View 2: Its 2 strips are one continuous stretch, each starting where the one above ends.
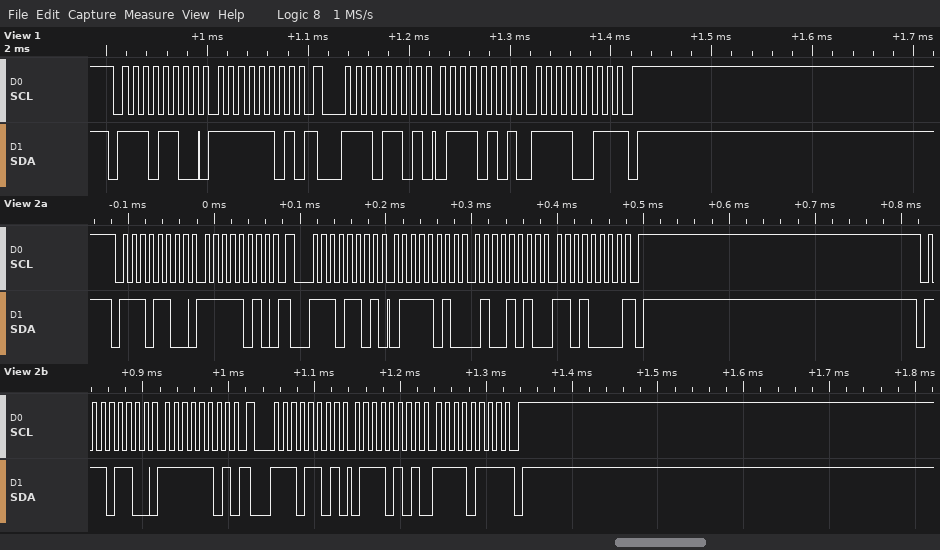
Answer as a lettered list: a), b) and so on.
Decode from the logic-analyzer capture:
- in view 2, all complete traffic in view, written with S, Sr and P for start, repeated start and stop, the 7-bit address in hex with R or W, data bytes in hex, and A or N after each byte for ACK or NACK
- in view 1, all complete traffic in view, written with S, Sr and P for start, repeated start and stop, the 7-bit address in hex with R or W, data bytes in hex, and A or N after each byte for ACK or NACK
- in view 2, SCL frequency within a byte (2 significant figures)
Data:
a) S 76W A FA A Sr 76R A 7A A 4A A D0 N P S 76W A FD A Sr 76R A 75 A F7 N P
b) S 76W A FD A Sr 76R A 75 A F3 N P
c) 100 kHz
